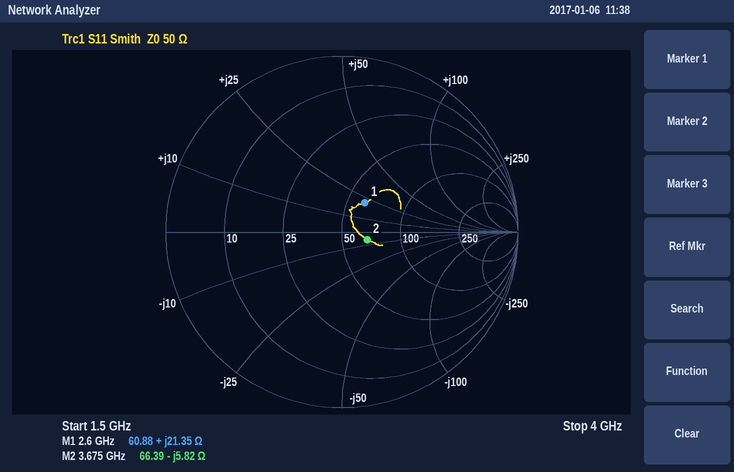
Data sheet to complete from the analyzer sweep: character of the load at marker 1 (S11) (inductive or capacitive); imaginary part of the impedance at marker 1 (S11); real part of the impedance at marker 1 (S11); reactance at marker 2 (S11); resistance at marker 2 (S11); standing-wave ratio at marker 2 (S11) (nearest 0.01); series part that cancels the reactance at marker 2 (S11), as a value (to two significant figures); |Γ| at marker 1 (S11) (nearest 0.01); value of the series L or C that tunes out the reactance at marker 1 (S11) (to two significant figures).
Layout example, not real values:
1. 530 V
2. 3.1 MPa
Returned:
1. inductive
2. +21.35 Ω
3. 60.88 Ω
4. -5.82 Ω
5. 66.39 Ω
6. 1.35
7. 250 pH
8. 0.21
9. 2.9 pF
